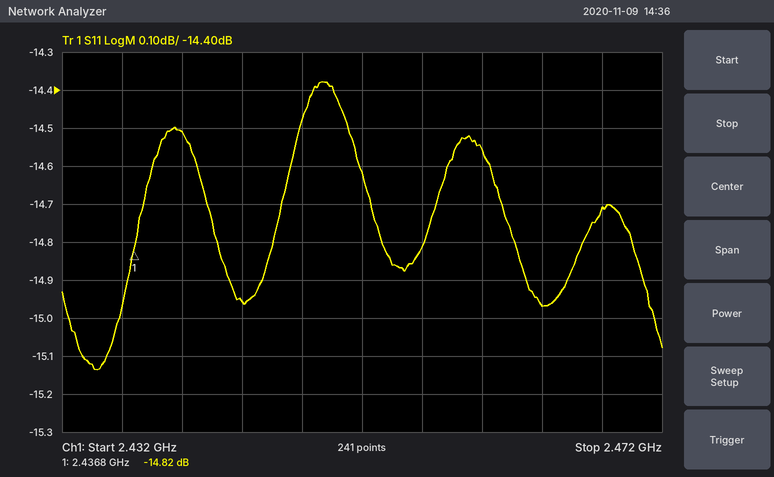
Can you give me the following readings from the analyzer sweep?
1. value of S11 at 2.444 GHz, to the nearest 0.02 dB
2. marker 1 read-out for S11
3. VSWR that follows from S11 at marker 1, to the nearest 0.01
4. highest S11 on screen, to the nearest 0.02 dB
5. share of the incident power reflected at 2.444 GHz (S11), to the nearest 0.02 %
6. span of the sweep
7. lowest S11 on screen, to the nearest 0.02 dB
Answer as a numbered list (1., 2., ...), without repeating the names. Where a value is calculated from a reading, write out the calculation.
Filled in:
1. -14.96 dB
2. -14.82 dB
3. (1 + 0.1816)/(1 − 0.1816) ≈ 1.44
4. -14.38 dB
5. 10^(-14.96/10) ≈ 3.19 %, so 3.20 % to the nearest 0.02 %
6. 40 MHz
7. -15.14 dB
